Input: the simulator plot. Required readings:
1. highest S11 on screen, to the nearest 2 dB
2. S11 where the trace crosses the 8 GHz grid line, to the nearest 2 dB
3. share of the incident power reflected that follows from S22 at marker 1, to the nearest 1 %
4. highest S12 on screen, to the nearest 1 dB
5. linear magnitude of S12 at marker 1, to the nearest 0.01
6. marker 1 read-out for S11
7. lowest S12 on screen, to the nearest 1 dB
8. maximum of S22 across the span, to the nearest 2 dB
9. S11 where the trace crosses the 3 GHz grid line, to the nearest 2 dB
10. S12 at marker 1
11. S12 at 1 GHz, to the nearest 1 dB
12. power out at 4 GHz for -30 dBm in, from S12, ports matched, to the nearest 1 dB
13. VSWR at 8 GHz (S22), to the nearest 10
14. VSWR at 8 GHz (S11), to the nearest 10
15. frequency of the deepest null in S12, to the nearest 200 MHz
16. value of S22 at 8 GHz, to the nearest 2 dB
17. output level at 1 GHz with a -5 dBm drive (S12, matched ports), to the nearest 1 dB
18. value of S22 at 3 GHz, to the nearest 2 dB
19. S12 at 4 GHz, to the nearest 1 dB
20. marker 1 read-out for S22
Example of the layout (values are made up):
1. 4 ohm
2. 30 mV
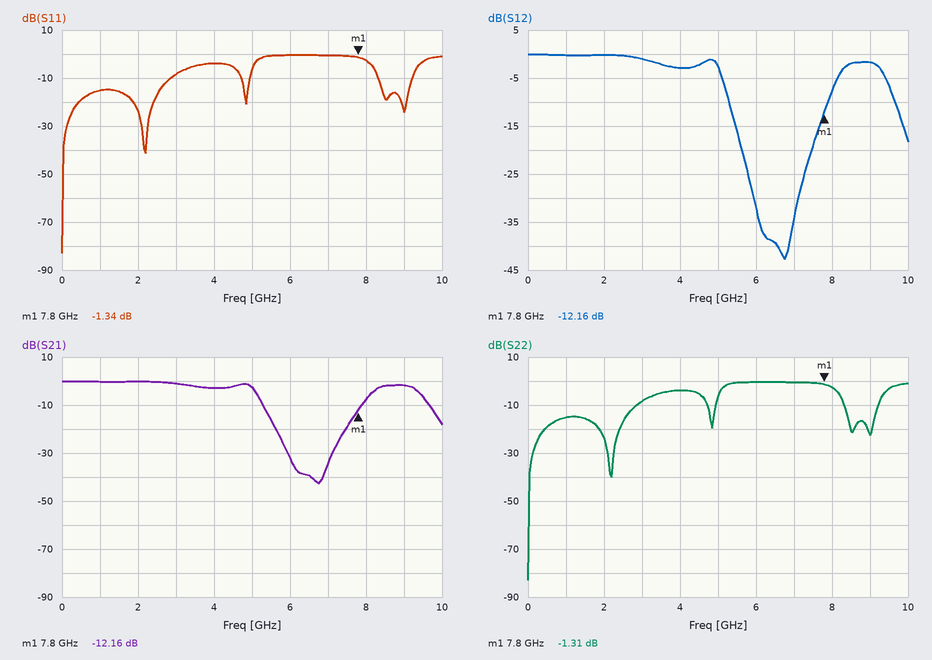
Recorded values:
1. 0 dB
2. -2 dB
3. 74 %
4. 0 dB
5. 0.25
6. -1.34 dB
7. -43 dB
8. 0 dB
9. -8 dB
10. -12.16 dB
11. 0 dB
12. -33 dBm
13. 10
14. 10
15. 6.8 GHz
16. -2 dB
17. -5 dBm
18. -8 dB
19. -3 dB
20. -1.31 dB
